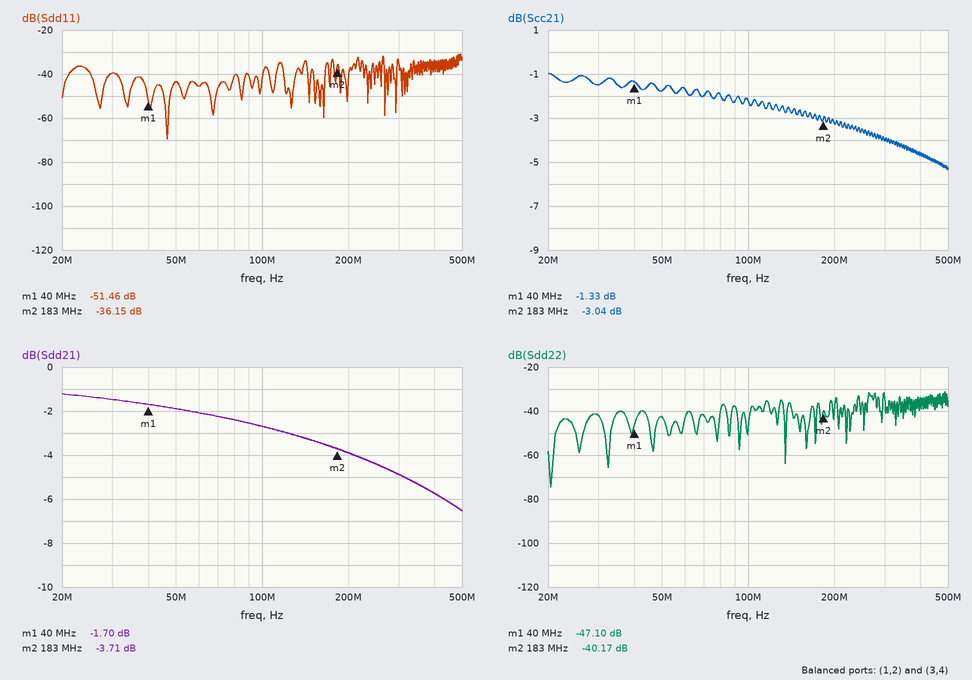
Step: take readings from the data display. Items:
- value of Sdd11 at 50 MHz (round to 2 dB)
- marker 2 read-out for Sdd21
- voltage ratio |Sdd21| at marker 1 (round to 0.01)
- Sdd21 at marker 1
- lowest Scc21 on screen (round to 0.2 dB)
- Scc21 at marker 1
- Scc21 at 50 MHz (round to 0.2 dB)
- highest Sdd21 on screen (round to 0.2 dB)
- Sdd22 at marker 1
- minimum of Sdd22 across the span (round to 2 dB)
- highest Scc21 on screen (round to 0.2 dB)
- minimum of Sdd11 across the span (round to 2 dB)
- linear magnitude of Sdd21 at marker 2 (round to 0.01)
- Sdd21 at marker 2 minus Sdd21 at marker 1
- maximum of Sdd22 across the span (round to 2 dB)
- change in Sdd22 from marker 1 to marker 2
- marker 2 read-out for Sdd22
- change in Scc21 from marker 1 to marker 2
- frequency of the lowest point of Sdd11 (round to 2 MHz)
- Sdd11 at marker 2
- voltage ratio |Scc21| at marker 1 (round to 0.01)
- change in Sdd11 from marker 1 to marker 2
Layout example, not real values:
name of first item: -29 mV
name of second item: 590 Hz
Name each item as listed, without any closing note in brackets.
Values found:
value of Sdd11 at 50 MHz: -44 dB
marker 2 read-out for Sdd21: -3.71 dB
voltage ratio |Sdd21| at marker 1: 0.82
Sdd21 at marker 1: -1.70 dB
lowest Scc21 on screen: -5.4 dB
Scc21 at marker 1: -1.33 dB
Scc21 at 50 MHz: -1.8 dB
highest Sdd21 on screen: -1.2 dB
Sdd22 at marker 1: -47.10 dB
minimum of Sdd22 across the span: -74 dB
highest Scc21 on screen: -1.0 dB
minimum of Sdd11 across the span: -70 dB
linear magnitude of Sdd21 at marker 2: 0.65
Sdd21 at marker 2 minus Sdd21 at marker 1: -2.01 dB
maximum of Sdd22 across the span: -32 dB
change in Sdd22 from marker 1 to marker 2: 6.93 dB
marker 2 read-out for Sdd22: -40.17 dB
change in Scc21 from marker 1 to marker 2: -1.71 dB
frequency of the lowest point of Sdd11: 46 MHz
Sdd11 at marker 2: -36.15 dB
voltage ratio |Scc21| at marker 1: 0.86
change in Sdd11 from marker 1 to marker 2: 15.31 dB
